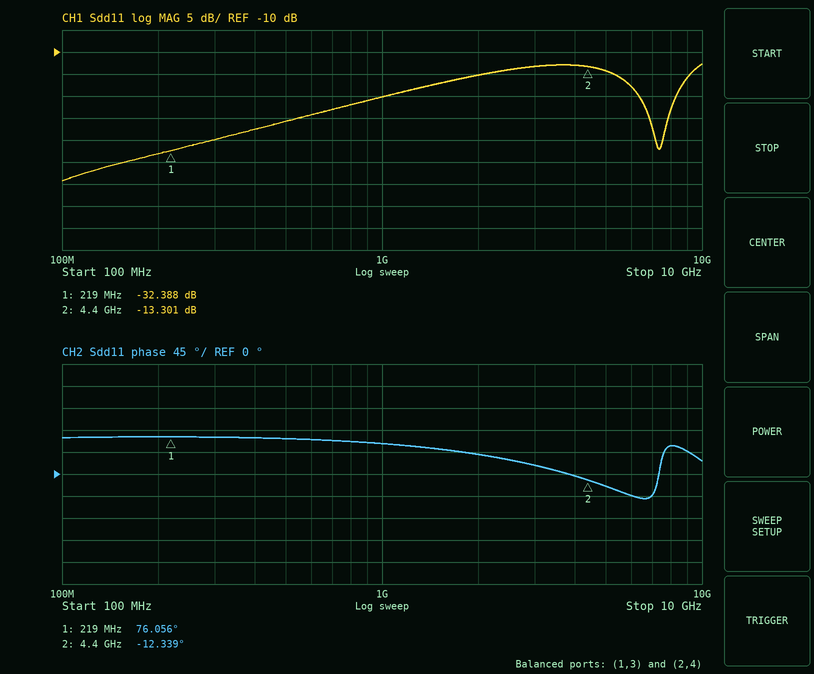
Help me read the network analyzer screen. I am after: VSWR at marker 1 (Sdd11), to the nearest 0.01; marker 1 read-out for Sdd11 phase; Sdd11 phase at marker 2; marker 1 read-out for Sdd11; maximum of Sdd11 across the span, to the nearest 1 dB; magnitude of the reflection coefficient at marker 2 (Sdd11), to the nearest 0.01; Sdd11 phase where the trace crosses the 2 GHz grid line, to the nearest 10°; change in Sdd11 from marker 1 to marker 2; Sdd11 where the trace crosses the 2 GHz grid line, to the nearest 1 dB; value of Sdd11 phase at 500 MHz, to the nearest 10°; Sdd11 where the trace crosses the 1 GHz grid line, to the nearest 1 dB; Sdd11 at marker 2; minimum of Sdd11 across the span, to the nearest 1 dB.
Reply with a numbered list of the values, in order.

1. 1.05
2. 76.056°
3. -12.339°
4. -32.388 dB
5. -13 dB
6. 0.22
7. 40°
8. 19.087 dB
9. -15 dB
10. 70°
11. -20 dB
12. -13.301 dB
13. -39 dB
